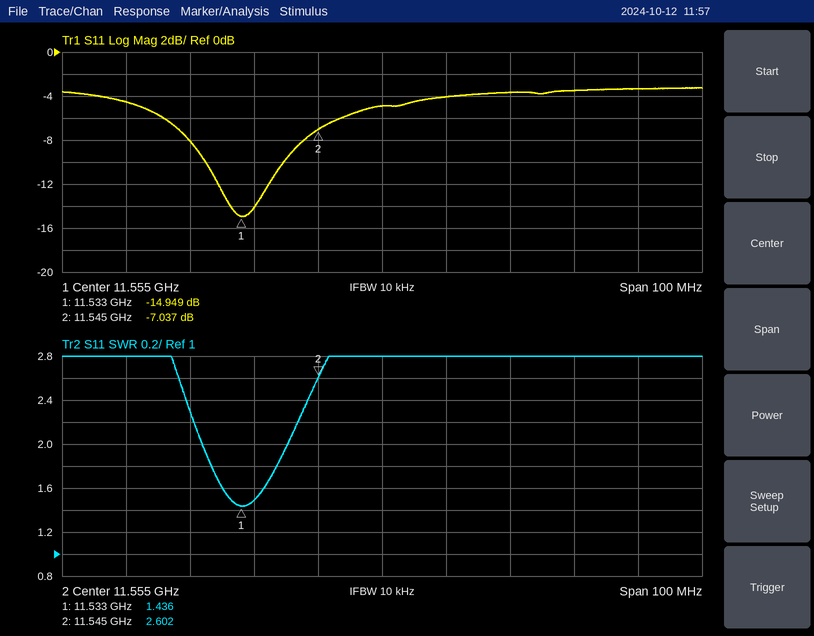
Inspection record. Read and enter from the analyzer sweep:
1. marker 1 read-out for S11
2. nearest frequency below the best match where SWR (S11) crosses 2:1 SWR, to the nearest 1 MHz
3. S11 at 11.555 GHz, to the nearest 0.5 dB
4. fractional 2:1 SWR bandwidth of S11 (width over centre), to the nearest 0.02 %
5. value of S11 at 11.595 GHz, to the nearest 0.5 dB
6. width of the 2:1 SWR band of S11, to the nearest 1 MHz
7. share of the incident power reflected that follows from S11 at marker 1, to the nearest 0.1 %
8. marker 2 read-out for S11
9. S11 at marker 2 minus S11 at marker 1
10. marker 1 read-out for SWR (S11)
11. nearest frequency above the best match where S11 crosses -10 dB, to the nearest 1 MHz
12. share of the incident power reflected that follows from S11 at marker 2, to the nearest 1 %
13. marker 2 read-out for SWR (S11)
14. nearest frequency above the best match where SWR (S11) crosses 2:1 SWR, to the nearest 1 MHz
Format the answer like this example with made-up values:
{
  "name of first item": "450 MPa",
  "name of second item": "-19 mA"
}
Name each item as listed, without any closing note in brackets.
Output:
{
  "marker 1 read-out for S11": "-14.949 dB",
  "nearest frequency below the best match where SWR (S11) crosses 2:1 SWR, to the nearest 1 MHz": "11.527 GHz",
  "S11 at 11.555 GHz, to the nearest 0.5 dB": "-5.0 dB",
  "fractional 2:1 SWR bandwidth of S11 (width over centre), to the nearest 0.02 %": "0.12 %",
  "value of S11 at 11.595 GHz, to the nearest 0.5 dB": "-3.5 dB",
  "width of the 2:1 SWR band of S11, to the nearest 1 MHz": "13 MHz",
  "share of the incident power reflected that follows from S11 at marker 1, to the nearest 0.1 %": "3.2 %",
  "marker 2 read-out for S11": "-7.037 dB",
  "S11 at marker 2 minus S11 at marker 1": "7.912 dB",
  "marker 1 read-out for SWR": "1.436",
  "nearest frequency above the best match where S11 crosses -10 dB, to the nearest 1 MHz": "11.540 GHz",
  "share of the incident power reflected that follows from S11 at marker 2, to the nearest 1 %": "20 %",
  "marker 2 read-out for SWR": "2.602",
  "nearest frequency above the best match where SWR (S11) crosses 2:1 SWR, to the nearest 1 MHz": "11.540 GHz"
}
